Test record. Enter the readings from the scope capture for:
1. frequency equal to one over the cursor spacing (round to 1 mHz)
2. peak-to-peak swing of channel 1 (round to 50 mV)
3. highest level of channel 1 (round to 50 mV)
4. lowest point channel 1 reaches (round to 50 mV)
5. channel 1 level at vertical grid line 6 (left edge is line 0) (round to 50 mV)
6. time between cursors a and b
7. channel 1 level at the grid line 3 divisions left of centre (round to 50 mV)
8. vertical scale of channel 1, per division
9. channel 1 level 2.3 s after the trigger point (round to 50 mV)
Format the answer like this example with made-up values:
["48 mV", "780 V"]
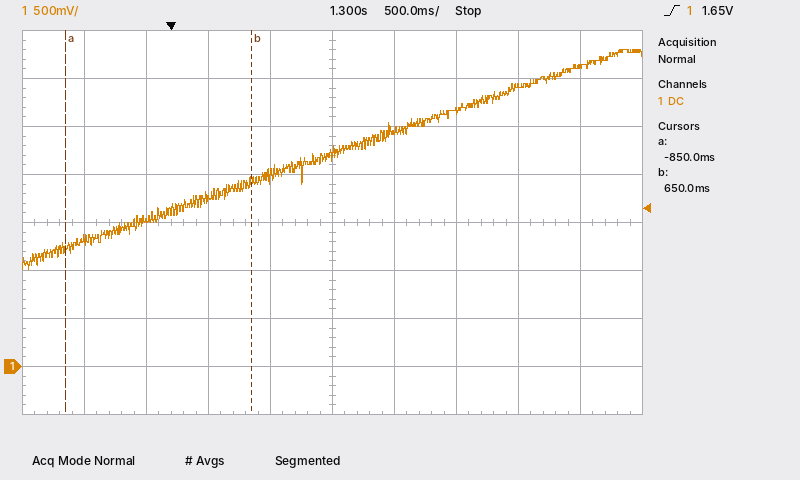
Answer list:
["667 mHz", "2.30 V", "3.30 V", "1.00 V", "2.45 V", "1.50 s", "1.55 V", "500 mV", "2.65 V"]
